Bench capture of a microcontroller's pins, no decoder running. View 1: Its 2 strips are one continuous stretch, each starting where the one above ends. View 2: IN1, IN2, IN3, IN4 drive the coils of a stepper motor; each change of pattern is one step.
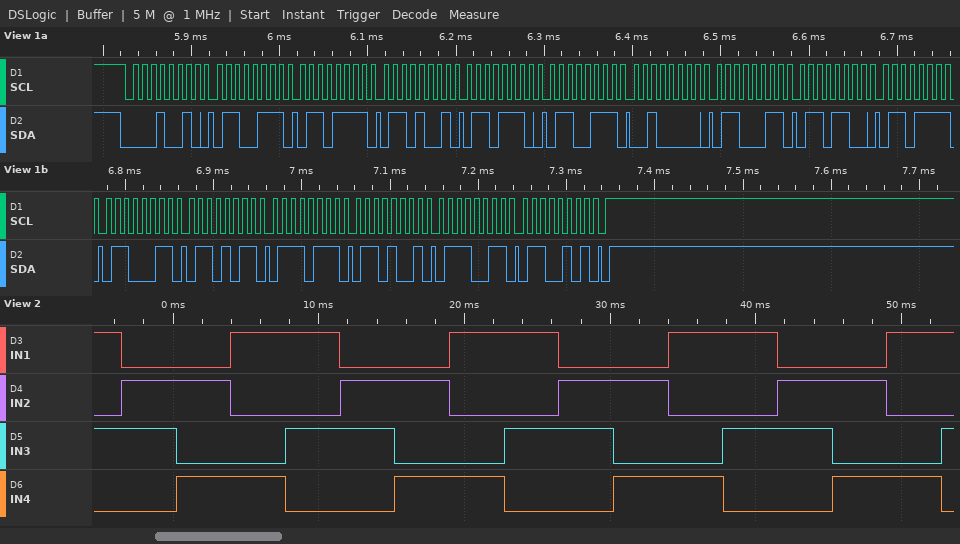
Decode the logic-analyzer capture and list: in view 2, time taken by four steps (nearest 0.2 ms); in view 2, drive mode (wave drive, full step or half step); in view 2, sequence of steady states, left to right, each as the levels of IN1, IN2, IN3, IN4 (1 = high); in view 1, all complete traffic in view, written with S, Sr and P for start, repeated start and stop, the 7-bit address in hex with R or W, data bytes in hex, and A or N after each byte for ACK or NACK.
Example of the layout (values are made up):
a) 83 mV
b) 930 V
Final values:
a) 15.0 ms
b) full step
c) 1010 0110 0101 1001 1010 0110 0101 1001 1010 0110 0101 1001 1010 0110 0101 1001 1010
d) S 09W A 67 A 6F A 69 A 6E A 67 A 20 A 63 A 6C A 6F A 63 A 6B A 77 A 69 A 73 A 65 A P
